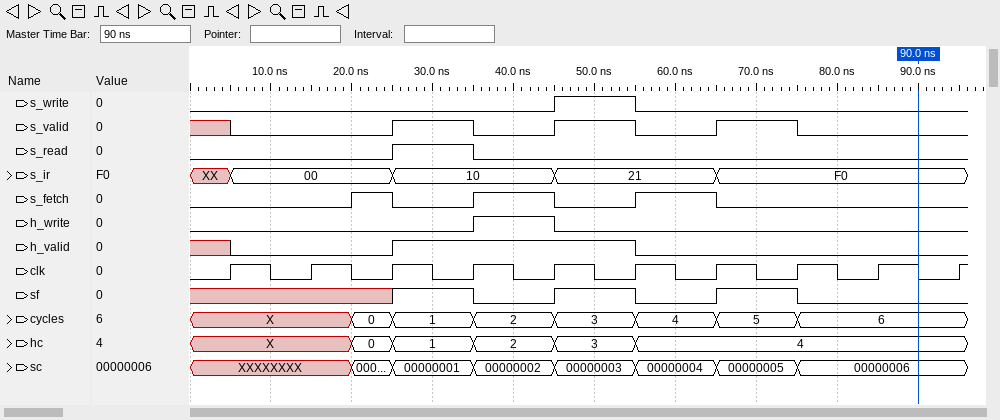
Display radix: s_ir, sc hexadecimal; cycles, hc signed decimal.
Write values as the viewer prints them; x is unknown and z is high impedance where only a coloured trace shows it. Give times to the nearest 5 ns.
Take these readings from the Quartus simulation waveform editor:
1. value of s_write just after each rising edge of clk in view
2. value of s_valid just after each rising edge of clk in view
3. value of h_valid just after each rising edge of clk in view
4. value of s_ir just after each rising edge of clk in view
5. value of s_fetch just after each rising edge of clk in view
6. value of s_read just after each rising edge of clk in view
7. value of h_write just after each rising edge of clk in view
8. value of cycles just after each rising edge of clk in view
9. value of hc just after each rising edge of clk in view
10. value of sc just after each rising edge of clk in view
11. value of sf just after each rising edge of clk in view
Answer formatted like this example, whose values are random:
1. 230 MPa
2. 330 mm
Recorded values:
1. 0 0 0 0 1 0 0 0 0 0
2. 0 0 1 0 1 0 1 0 0 0
3. 0 0 1 1 1 0 0 0 0 0
4. 00, 00, 10, 10, 21, 21, F0, F0, F0, F0
5. 0 0 0 1 0 1 0 0 0 0
6. 0 0 1 0 0 0 0 0 0 0
7. 0 0 0 1 0 0 0 0 0 0
8. X, X, 1, 2, 3, 4, 5, 6, 6, 6
9. X, X, 1, 2, 3, 4, 4, 4, 4, 4
10. XXXXXXXX, XXXXXXXX, 00000001, 00000002, 00000003, 00000004, 00000005, 00000006, 00000006, 00000006
11. x x 1 0 1 0 1 0 0 0
